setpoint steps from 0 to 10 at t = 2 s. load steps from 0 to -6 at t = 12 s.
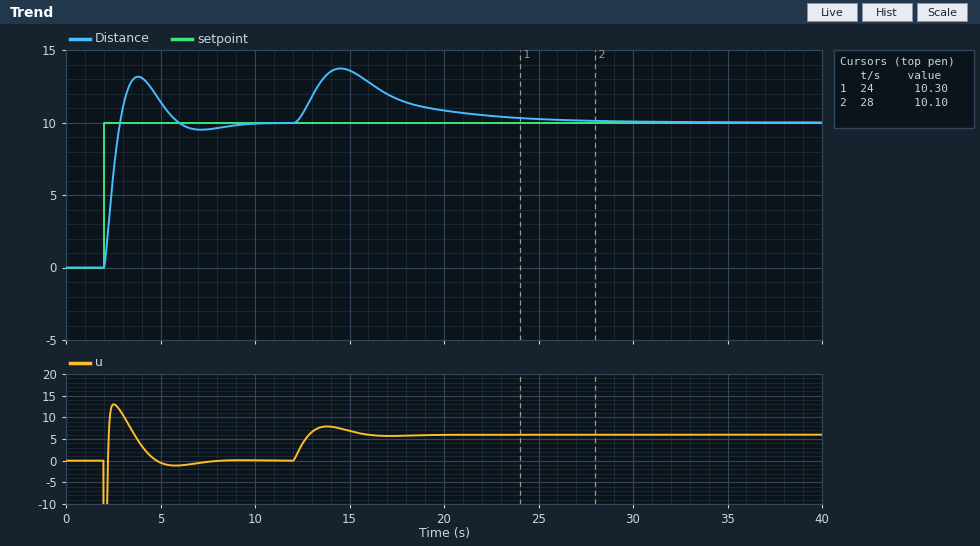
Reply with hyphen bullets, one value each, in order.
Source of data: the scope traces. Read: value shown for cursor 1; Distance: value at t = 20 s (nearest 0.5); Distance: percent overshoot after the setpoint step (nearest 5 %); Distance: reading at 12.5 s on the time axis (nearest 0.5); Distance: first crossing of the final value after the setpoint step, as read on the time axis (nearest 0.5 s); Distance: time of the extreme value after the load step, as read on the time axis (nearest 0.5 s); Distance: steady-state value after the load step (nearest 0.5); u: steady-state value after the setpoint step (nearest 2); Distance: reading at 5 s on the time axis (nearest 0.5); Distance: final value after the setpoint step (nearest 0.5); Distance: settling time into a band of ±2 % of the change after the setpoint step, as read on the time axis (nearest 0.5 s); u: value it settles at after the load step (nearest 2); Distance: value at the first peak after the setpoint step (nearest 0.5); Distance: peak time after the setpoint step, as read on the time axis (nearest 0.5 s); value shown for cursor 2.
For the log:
- 10.30
- 11.0
- 30 %
- 10.5
- 3.0 s
- 14.5 s
- 10.0
- 0
- 11.5
- 10.0
- 9.0 s
- 6
- 13.0
- 4.0 s
- 10.10
